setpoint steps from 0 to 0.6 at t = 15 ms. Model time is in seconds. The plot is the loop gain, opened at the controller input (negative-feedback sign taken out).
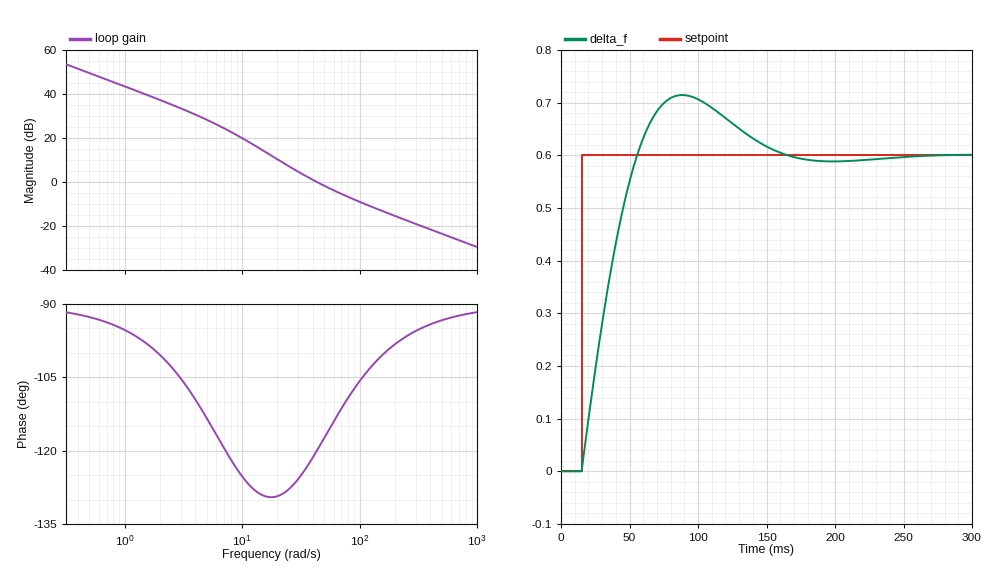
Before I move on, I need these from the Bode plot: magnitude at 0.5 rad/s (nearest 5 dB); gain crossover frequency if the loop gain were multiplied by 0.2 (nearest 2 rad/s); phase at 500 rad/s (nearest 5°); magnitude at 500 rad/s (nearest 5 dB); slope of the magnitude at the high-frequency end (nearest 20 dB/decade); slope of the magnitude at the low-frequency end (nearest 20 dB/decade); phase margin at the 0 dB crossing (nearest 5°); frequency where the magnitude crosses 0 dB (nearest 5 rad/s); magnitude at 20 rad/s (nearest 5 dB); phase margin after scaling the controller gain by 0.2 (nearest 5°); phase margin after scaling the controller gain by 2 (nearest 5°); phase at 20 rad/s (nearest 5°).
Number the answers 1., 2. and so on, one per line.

1. 50 dB
2. 16 rad/s
3. -95°
4. -25 dB
5. -20 dB/decade
6. -20 dB/decade
7. 60°
8. 45 rad/s
9. 10 dB
10. 50°
11. 70°
12. -130°
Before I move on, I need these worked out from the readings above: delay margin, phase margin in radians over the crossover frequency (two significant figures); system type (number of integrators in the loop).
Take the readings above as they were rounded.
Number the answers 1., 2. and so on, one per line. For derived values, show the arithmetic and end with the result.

1. 60 × π / 180 / 45 = 0.023 s
2. 1
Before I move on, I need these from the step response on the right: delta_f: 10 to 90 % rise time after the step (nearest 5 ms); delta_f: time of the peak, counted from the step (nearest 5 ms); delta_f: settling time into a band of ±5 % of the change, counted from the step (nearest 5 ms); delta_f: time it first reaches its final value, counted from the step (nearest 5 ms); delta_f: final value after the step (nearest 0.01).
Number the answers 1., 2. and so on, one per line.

1. 30 ms
2. 75 ms
3. 125 ms
4. 40 ms
5. 0.60
